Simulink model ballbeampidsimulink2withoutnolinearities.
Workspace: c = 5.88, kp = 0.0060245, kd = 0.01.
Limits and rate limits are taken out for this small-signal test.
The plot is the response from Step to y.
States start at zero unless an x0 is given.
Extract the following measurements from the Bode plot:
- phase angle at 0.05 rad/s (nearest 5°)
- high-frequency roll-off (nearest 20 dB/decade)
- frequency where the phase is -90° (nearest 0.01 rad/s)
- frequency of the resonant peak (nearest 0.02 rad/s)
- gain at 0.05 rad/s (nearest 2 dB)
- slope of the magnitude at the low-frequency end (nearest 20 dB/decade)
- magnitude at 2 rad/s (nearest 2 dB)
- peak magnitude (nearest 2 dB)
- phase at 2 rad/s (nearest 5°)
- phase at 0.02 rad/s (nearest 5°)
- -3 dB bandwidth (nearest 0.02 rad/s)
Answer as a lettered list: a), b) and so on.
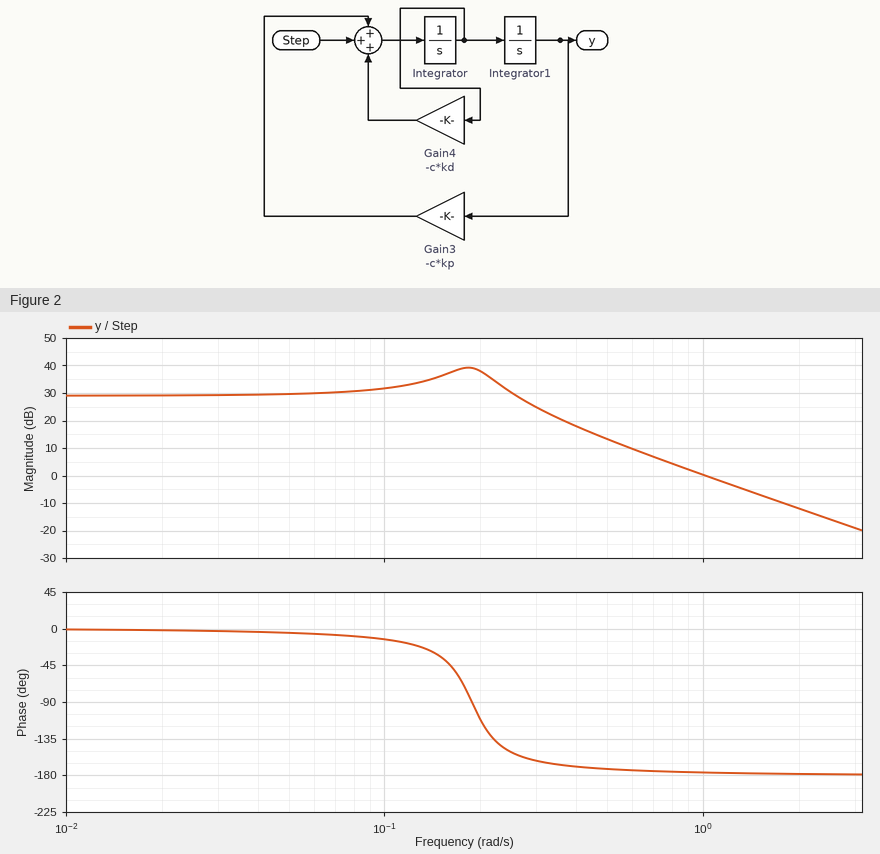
a) -5°
b) -40 dB/decade
c) 0.19 rad/s
d) 0.18 rad/s
e) 30 dB
f) 0 dB/decade
g) -12 dB
h) 40 dB
i) -180°
j) 0°
k) 0.28 rad/s
